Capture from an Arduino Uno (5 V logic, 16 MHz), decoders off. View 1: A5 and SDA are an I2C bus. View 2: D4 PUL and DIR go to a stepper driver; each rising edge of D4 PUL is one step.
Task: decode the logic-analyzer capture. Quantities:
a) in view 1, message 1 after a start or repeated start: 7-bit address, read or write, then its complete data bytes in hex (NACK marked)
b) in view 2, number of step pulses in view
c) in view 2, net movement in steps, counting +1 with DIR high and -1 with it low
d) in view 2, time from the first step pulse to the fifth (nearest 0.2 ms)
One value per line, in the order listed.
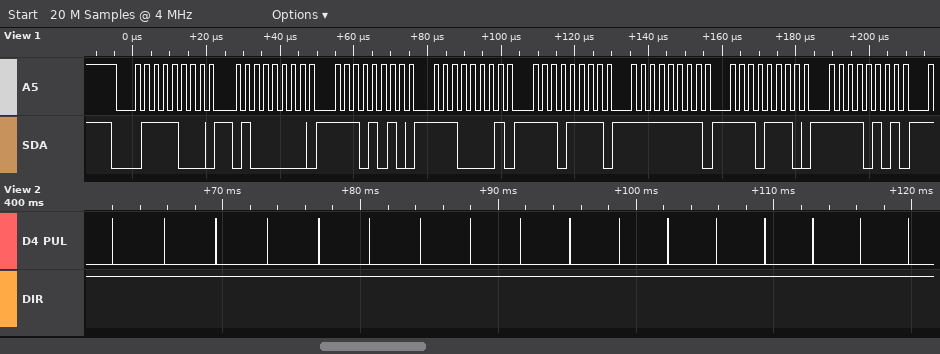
0x3C write: 40 EA E1 EF FF EE F5
17
+17
15.0 ms
